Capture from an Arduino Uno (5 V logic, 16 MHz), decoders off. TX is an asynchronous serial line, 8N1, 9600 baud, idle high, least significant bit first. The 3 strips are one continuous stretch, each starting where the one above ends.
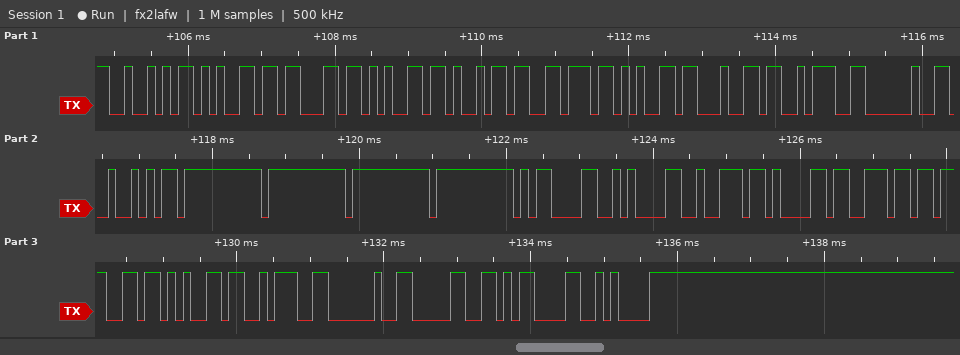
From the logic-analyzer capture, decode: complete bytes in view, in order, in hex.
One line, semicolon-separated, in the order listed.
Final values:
52 65 63 65 69 76 65 64 3A 20 52 FF FF FF FF 0D 0A 72 61 6E 67 65 3A 20 30 0D 0A
